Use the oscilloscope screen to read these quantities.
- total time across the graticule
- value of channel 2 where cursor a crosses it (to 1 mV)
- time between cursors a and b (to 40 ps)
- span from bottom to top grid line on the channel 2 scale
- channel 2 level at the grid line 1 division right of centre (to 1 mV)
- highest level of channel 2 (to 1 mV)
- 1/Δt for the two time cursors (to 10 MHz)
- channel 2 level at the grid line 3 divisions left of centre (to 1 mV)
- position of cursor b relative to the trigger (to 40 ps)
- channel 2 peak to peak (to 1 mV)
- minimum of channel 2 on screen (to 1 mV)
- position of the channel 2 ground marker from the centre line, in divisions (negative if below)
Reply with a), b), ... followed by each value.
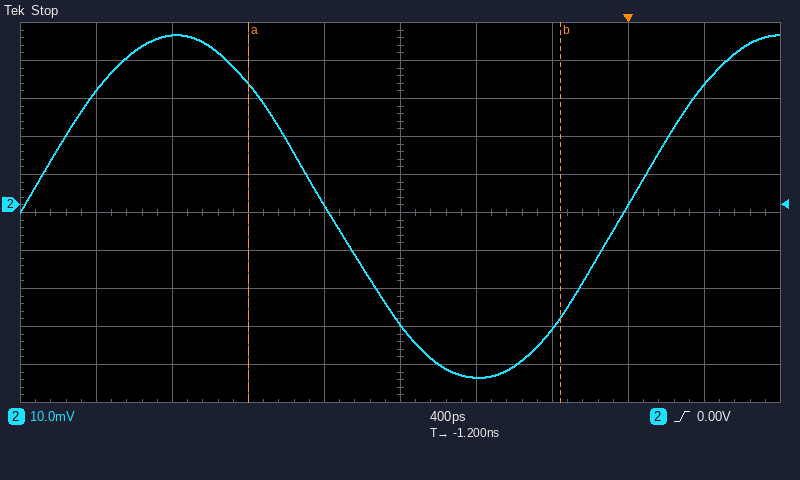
a) 4 ns
b) 32 mV
c) 1.64 ns
d) 100 mV
e) -45 mV
f) 45 mV
g) 610 MHz
h) 45 mV
i) -360 ps
j) 90 mV
k) -45 mV
l) +0.2 div
